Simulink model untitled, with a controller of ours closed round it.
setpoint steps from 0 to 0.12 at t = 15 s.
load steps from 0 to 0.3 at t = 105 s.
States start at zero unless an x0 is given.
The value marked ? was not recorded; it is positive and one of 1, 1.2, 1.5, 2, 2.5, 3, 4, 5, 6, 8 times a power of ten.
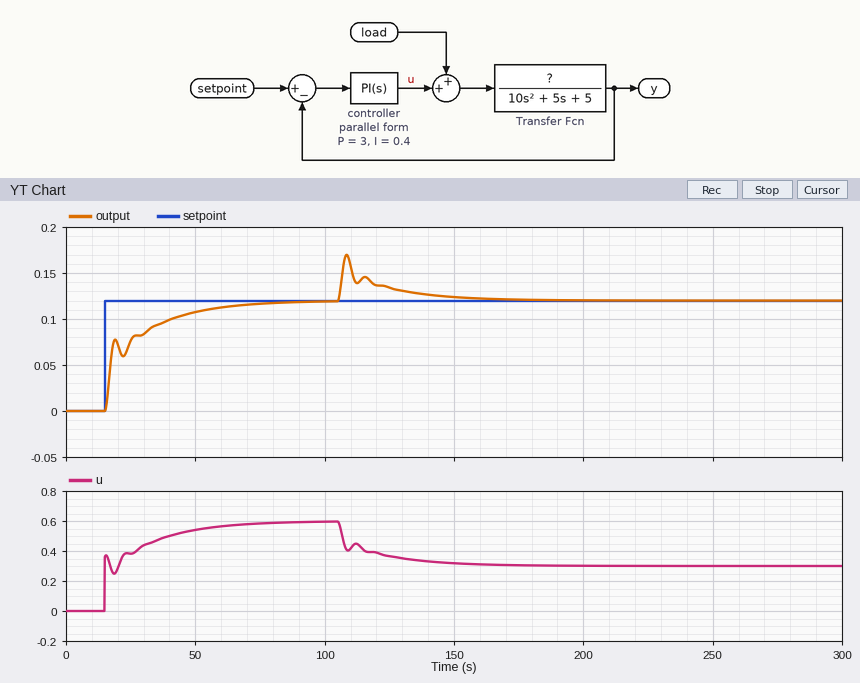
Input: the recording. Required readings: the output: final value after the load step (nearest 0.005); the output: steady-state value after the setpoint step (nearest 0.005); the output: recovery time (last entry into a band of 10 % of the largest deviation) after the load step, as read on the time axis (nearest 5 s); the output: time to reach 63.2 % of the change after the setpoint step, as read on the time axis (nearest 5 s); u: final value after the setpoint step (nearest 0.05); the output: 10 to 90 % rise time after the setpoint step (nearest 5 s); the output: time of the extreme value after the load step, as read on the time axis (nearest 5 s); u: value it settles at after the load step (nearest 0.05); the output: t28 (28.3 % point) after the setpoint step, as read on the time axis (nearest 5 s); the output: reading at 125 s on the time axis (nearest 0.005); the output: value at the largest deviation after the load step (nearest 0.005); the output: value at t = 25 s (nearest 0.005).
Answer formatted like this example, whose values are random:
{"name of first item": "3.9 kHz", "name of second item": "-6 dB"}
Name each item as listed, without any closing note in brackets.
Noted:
{"the output: final value after the load step": "0.120", "the output: steady-state value after the setpoint step": "0.120", "the output: recovery time (last entry into a band of 10 % of the largest deviation) after the load step, as read on the time axis": "145 s", "the output: time to reach 63.2 % of the change after the setpoint step, as read on the time axis": "20 s", "u: final value after the setpoint step": "0.60", "the output: 10 to 90 % rise time after the setpoint step": "35 s", "the output: time of the extreme value after the load step, as read on the time axis": "110 s", "u: value it settles at after the load step": "0.30", "the output: t28 (28.3 % point) after the setpoint step, as read on the time axis": "15 s", "the output: reading at 125 s on the time axis": "0.135", "the output: value at the largest deviation after the load step": "0.170", "the output: value at t = 25 s": "0.075"}
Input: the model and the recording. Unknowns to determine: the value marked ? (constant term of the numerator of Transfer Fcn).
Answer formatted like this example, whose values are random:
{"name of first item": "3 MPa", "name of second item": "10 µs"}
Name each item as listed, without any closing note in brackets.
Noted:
{"the value marked ?": "1"}
